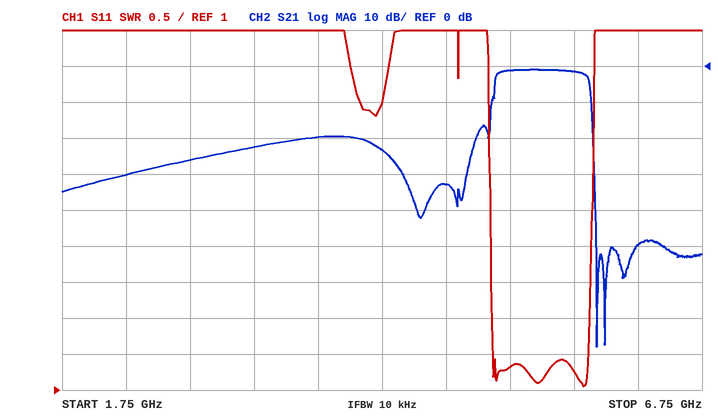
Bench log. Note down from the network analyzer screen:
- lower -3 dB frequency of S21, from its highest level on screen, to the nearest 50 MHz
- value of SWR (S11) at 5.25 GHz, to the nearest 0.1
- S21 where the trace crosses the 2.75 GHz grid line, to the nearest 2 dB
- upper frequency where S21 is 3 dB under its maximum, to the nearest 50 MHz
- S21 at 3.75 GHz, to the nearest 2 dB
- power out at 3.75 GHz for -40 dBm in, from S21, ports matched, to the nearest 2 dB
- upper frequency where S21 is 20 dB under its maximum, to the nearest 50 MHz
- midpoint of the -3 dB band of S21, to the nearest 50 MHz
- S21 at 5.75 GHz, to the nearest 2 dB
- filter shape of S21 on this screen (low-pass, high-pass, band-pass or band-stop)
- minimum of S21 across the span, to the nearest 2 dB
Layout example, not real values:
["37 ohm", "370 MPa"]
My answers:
["5.15 GHz", "1.3", "-26 dB", "5.85 GHz", "-20 dB", "-60 dBm", "5.90 GHz", "5.50 GHz", "-2 dB", "band-pass", "-78 dB"]
